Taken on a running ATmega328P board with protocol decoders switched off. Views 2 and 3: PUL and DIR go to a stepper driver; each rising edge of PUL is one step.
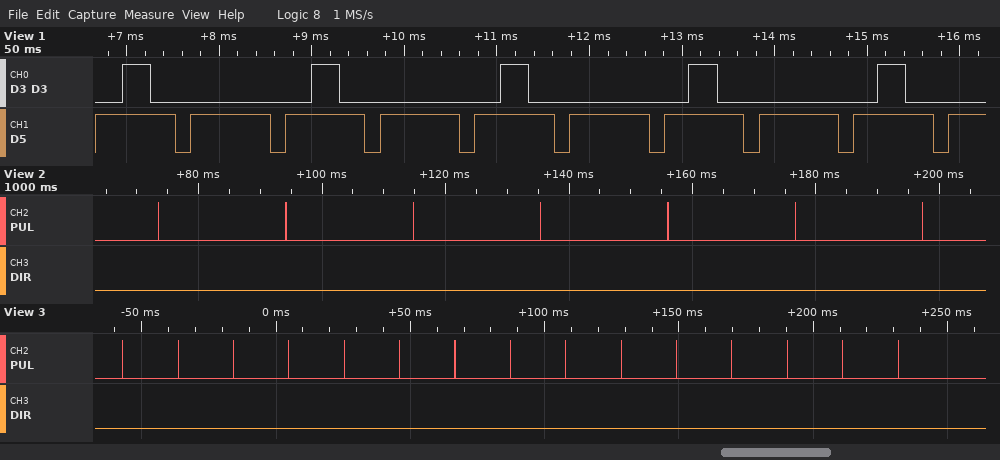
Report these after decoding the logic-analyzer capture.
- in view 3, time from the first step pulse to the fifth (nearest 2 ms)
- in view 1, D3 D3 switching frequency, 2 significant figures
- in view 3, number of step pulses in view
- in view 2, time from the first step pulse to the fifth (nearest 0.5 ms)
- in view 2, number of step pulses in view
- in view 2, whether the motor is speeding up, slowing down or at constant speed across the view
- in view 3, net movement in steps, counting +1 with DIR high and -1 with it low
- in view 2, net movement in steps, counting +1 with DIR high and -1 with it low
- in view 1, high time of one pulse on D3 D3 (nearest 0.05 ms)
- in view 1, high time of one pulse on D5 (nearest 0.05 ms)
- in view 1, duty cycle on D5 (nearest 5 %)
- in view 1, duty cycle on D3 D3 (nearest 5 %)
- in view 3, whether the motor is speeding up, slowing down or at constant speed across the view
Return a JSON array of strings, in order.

["82 ms", "490 Hz", "15", "82.5 ms", "7", "constant speed", "-15", "-7", "0.30 ms", "0.85 ms", "85 %", "15 %", "constant speed"]
